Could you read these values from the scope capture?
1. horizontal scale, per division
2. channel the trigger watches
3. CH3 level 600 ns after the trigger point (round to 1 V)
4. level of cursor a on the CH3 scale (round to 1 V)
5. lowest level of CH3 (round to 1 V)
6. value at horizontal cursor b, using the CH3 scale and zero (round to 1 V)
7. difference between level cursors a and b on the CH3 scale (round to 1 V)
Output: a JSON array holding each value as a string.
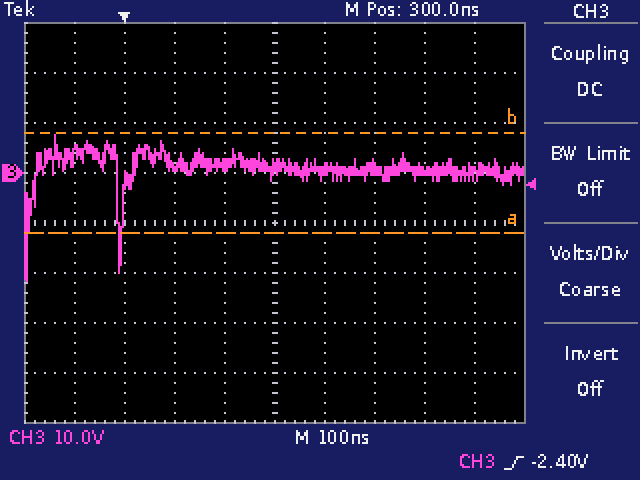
["100 ns", "CH3", "0 V", "-12 V", "-22 V", "8 V", "20 V"]
